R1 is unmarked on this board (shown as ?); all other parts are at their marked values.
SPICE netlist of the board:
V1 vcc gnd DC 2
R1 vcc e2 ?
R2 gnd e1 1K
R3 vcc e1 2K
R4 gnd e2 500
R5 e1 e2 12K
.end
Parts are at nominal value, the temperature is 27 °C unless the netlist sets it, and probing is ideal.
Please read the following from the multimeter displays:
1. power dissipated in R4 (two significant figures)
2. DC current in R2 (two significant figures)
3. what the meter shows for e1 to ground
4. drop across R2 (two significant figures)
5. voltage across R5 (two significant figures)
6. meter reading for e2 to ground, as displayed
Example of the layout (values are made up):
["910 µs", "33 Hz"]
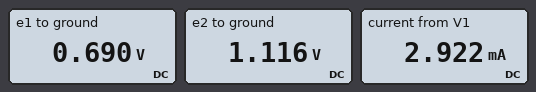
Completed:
["2.5 mW", "690 µA", "0.690 V", "690 mV", "430 mV", "1.116 V"]
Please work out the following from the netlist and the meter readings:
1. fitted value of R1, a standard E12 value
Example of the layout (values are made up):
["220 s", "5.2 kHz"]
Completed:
["390 Ω"]
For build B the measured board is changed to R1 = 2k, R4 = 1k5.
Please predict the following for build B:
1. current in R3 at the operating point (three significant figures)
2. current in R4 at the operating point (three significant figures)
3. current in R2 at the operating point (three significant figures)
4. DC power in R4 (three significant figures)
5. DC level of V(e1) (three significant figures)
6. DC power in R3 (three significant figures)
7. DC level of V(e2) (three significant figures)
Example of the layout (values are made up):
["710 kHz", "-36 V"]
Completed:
["662 µA", "563 µA", "676 µA", "476 µW", "676 mV", "876 µW", "845 mV"]
